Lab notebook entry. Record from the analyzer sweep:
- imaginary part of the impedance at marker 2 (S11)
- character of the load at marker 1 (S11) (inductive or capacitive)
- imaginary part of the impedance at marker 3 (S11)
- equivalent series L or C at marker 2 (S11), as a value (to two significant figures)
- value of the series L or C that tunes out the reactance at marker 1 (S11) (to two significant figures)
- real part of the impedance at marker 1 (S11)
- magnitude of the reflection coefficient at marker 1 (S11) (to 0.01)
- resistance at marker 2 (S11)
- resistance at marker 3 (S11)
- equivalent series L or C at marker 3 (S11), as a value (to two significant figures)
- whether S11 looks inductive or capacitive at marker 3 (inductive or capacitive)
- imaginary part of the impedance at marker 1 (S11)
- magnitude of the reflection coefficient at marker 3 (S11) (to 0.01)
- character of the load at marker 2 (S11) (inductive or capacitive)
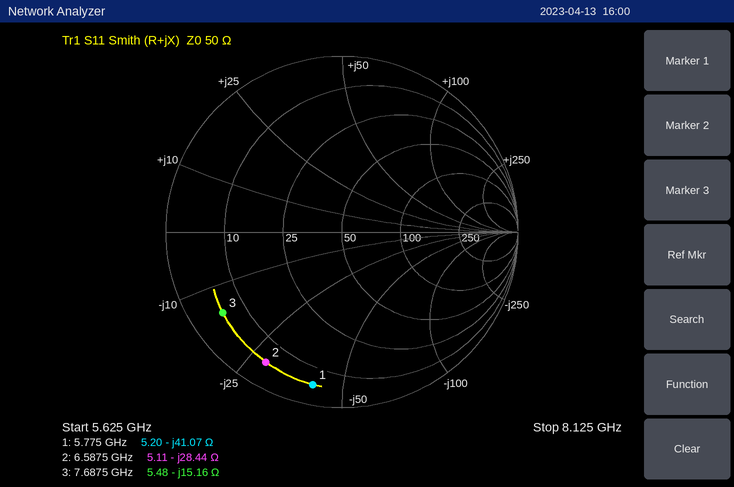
-28.44 Ω
capacitive
-15.16 Ω
850 fF
1.1 nH
5.20 Ω
0.88
5.11 Ω
5.48 Ω
1.4 pF
capacitive
-41.07 Ω
0.82
capacitive
